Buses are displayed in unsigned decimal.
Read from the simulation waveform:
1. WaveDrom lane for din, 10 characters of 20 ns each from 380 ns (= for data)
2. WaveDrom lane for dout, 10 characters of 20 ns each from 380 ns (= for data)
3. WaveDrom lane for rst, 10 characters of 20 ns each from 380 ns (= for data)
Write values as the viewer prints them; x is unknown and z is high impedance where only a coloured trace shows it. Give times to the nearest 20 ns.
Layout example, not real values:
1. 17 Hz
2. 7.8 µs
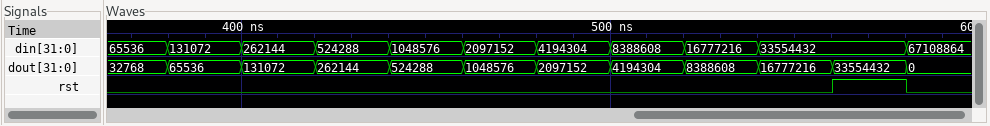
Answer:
1. {name: 'din', wave: '=========.', data: '131072 262144 524288 1048576 2097152 4194304 8388608 16777216 33554432'}
2. {name: 'dout', wave: '==========', data: '65536 131072 262144 524288 1048576 2097152 4194304 8388608 16777216 33554432'}
3. {name: 'rst', wave: '0........1'}
